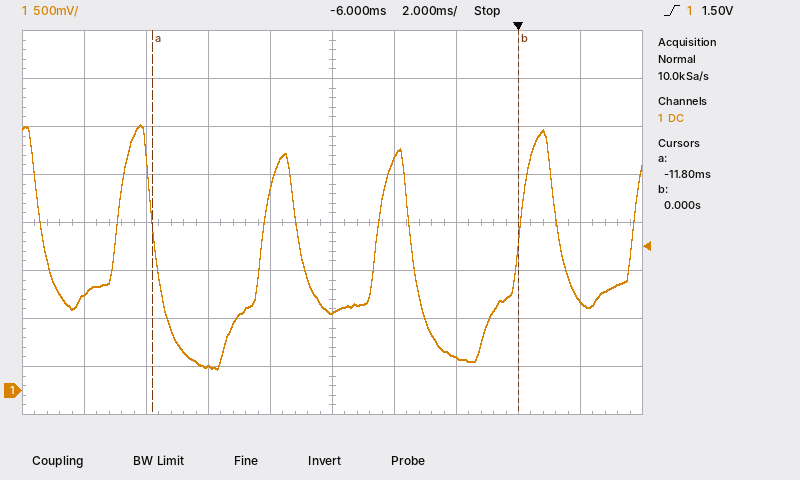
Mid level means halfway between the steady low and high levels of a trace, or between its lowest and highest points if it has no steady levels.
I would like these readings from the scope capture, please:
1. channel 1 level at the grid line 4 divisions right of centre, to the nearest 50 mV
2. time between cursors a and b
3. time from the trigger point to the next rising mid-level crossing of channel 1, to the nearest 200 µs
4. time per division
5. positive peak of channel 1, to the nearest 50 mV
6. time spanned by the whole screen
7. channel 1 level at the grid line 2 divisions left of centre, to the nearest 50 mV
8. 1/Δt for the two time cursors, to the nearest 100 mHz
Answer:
950 mV
11.8 ms
3.6 ms
2 ms
2.75 V
20 ms
250 mV
84.7 Hz
